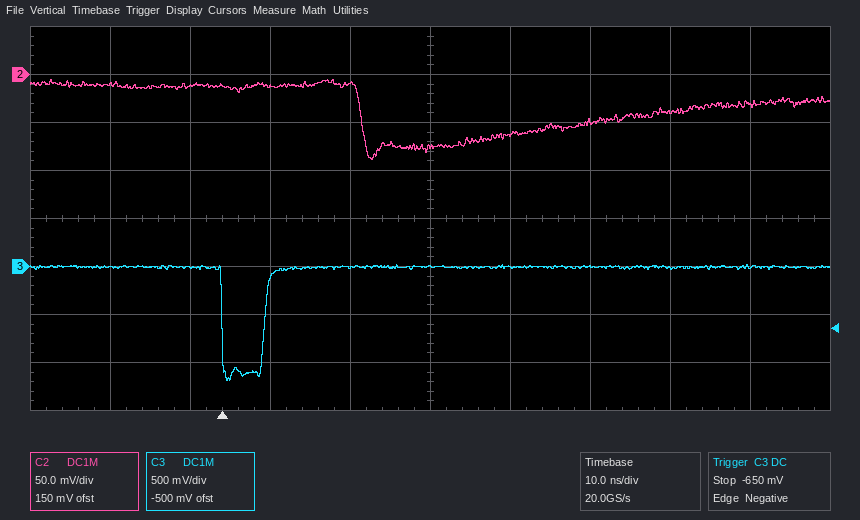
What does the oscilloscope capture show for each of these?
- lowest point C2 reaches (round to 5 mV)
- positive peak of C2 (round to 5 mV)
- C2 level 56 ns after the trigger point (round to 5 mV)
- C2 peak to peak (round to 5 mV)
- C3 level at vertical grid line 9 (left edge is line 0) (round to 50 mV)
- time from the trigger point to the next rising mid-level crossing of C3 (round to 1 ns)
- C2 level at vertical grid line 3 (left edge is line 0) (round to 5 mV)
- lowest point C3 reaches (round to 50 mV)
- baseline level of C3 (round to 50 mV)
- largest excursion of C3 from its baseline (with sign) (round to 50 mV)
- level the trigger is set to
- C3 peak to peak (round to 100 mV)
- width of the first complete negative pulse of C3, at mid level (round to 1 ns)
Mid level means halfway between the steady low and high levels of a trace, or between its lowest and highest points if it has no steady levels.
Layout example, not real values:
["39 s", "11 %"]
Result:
["-90 mV", "-5 mV", "-40 mV", "85 mV", "0 mV", "5 ns", "-10 mV", "-1.20 V", "0 mV", "-1.20 V", "-650 mV", "1.20 V", "5 ns"]
